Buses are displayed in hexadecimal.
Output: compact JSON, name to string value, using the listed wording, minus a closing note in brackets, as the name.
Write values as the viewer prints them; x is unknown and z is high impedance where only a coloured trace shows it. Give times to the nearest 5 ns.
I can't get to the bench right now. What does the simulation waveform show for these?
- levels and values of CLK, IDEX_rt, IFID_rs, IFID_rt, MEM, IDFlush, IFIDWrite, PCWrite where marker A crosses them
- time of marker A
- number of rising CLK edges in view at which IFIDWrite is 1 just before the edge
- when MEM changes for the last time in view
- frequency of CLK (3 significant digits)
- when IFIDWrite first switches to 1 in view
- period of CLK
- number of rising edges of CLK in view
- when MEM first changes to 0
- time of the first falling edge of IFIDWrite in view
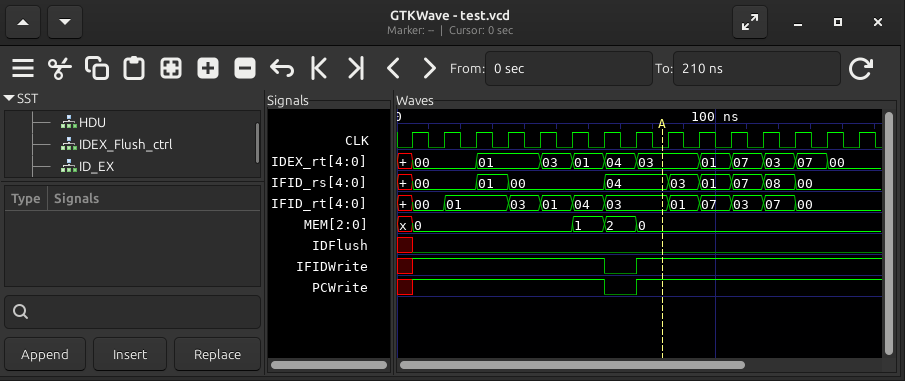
{"levels and values of CLK, IDEX_rt, IFID_rs, IFID_rt, MEM, IDFlush, IFIDWrite, PCWrite where marker A crosses them": "CLK=0, IDEX_rt=03, IFID_rs=04, IFID_rt=03, MEM=0, IDFlush=0, IFIDWrite=1, PCWrite=1", "time of marker A": "85 ns", "number of rising CLK edges in view at which IFIDWrite is 1 just before the edge": "13", "when MEM changes for the last time in view": "75 ns", "frequency of CLK": "100 MHz", "when IFIDWrite first switches to 1 in view": "5 ns", "period of CLK": "10 ns", "number of rising edges of CLK in view": "15", "when MEM first changes to 0": "5 ns", "time of the first falling edge of IFIDWrite in view": "65 ns"}
